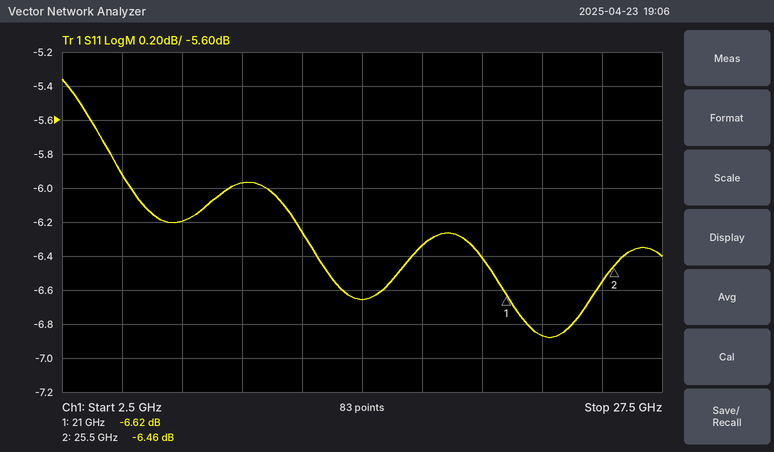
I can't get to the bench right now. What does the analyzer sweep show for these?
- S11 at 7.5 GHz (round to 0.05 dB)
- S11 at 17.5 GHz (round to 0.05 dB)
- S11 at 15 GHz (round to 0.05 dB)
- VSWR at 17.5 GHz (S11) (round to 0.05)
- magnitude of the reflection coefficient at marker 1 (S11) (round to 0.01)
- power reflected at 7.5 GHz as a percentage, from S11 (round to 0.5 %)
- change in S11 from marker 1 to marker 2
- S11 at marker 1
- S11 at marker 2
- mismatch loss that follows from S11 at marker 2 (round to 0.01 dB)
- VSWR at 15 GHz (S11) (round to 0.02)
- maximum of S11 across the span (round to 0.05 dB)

-6.20 dB
-6.35 dB
-6.65 dB
2.85
0.47
24.0 %
0.16 dB
-6.62 dB
-6.46 dB
1.11 dB
2.74
-5.35 dB
